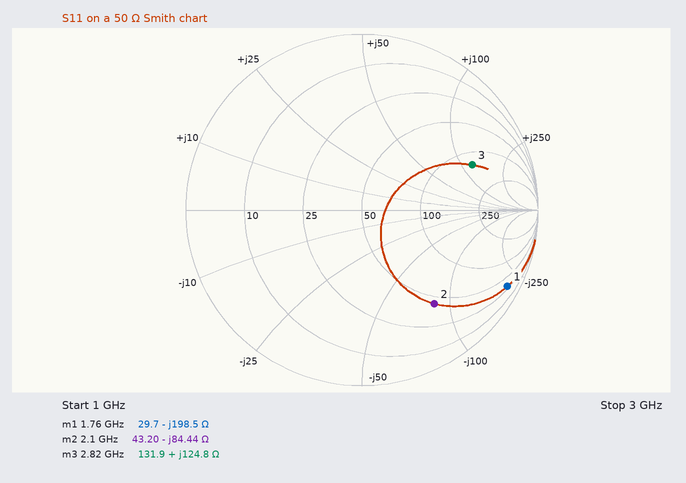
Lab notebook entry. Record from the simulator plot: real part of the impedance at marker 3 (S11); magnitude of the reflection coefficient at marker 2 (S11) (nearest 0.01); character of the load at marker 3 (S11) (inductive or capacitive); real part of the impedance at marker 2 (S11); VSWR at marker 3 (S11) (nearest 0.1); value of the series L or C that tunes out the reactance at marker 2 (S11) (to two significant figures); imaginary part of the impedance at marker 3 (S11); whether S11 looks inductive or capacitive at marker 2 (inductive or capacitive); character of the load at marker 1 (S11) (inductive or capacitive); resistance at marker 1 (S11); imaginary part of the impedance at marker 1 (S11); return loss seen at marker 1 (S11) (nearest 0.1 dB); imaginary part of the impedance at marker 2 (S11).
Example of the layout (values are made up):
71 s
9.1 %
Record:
131.9 Ω
0.67
inductive
43.20 Ω
5.2
6.4 nH
+124.8 Ω
capacitive
capacitive
29.7 Ω
-198.5 Ω
0.6 dB
-84.44 Ω
